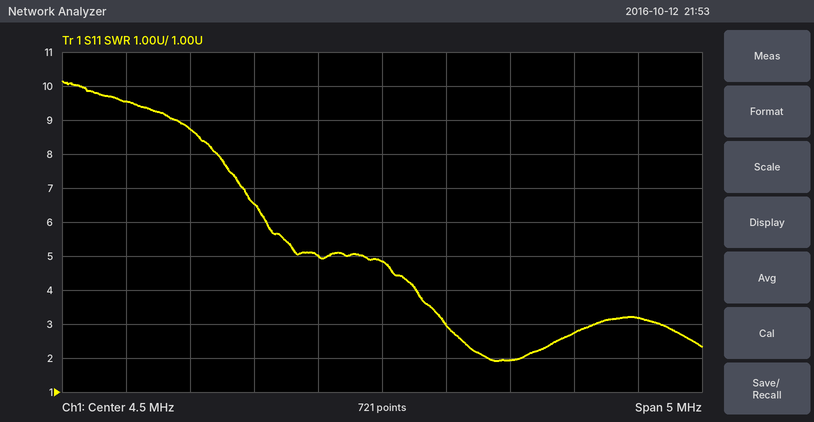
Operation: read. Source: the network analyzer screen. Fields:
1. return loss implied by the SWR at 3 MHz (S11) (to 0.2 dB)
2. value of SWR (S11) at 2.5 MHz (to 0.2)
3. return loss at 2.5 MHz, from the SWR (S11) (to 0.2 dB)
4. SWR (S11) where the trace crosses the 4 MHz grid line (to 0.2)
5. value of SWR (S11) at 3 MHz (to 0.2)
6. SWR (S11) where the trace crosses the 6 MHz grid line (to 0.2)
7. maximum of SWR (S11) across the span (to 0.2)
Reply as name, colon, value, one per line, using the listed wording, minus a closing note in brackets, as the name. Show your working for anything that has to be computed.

return loss implied by the SWR at 3 MHz (S11): −20 log10((8.8 − 1)/(8.8 + 1)) ≈ 2.0 dB
value of SWR (S11) at 2.5 MHz: 9.6
return loss at 2.5 MHz, from the SWR (S11): −20 log10((9.6 − 1)/(9.6 + 1)) ≈ 1.8 dB
SWR (S11) where the trace crosses the 4 MHz grid line: 5.0
value of SWR (S11) at 3 MHz: 8.8
SWR (S11) where the trace crosses the 6 MHz grid line: 2.8
maximum of SWR (S11) across the span: 10.2
